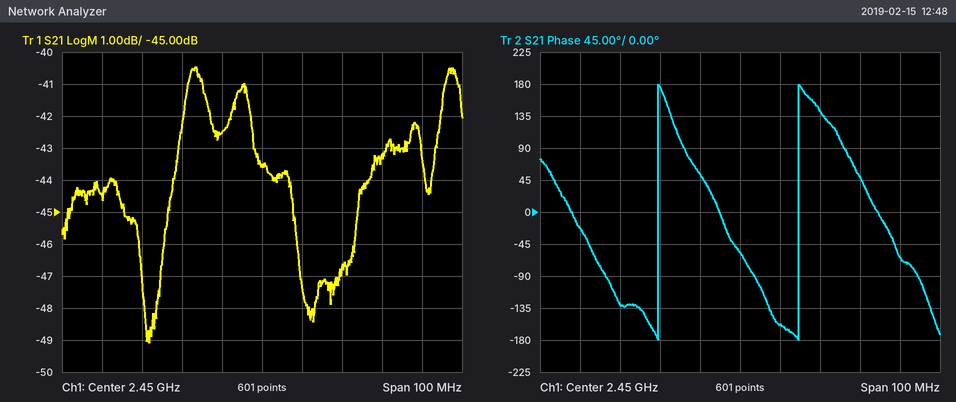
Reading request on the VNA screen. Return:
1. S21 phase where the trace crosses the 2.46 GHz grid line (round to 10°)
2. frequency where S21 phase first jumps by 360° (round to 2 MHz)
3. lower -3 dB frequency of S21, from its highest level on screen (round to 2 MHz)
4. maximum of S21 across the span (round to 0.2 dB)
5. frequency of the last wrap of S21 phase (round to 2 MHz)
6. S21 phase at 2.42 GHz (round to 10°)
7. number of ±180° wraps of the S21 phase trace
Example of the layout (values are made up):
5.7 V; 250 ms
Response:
-160°; 2.430 GHz; 2.428 GHz; -40.4 dB; 2.464 GHz; -130°; 2
